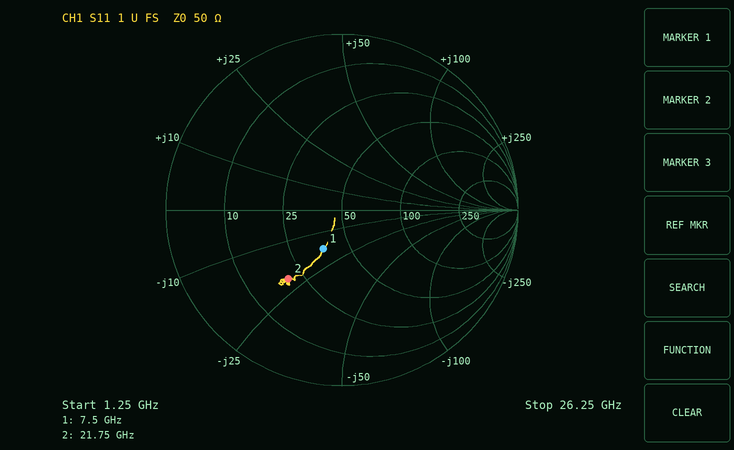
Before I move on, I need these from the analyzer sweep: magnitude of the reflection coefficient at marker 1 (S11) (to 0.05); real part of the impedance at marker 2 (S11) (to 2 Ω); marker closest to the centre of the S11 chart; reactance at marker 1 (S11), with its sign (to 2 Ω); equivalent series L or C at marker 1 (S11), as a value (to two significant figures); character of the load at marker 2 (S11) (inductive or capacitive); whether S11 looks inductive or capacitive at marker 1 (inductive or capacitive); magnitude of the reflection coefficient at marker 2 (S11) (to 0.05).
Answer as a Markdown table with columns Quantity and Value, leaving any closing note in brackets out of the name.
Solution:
| Quantity | Value |
|---|---|
| magnitude of the reflection coefficient at marker 1 (S11) | 0.25 |
| real part of the impedance at marker 2 (S11) | 20 Ω |
| marker closest to the centre of the S11 chart | marker 1 |
| reactance at marker 1 (S11), with its sign | -18 Ω |
| equivalent series L or C at marker 1 (S11), as a value | 1.2 pF |
| character of the load at marker 2 (S11) | capacitive |
| whether S11 looks inductive or capacitive at marker 1 | capacitive |
| magnitude of the reflection coefficient at marker 2 (S11) | 0.50 |
